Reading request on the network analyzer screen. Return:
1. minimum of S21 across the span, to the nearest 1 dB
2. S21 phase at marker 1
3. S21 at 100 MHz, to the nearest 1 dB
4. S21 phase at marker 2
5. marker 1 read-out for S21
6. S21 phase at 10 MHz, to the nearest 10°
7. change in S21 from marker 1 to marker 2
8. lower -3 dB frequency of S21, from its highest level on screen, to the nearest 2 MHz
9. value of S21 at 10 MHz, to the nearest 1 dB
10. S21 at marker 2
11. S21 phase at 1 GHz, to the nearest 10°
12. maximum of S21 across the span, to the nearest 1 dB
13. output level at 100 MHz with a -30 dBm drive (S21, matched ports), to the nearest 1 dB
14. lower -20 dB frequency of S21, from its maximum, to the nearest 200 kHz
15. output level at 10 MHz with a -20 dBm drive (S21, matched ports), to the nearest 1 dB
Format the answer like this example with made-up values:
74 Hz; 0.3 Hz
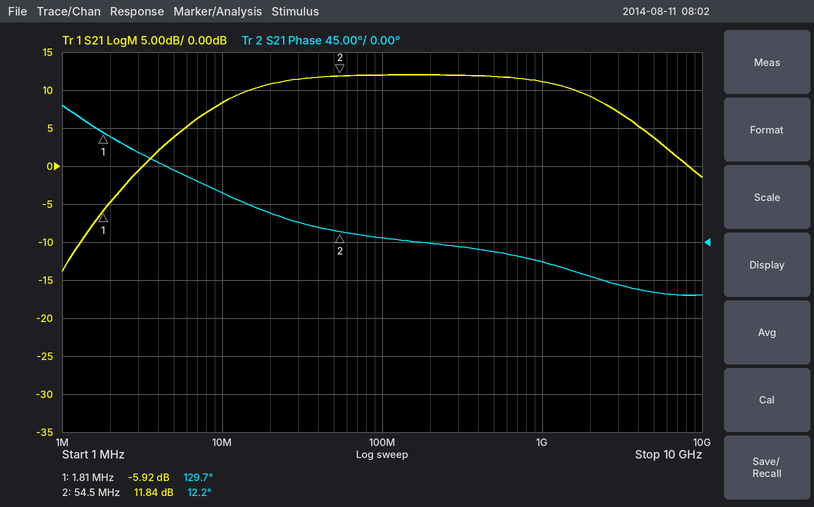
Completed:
-14 dB; 129.7°; 12 dB; 12.2°; -5.92 dB; 60°; 17.76 dB; 12 MHz; 8 dB; 11.84 dB; -20°; 12 dB; -18 dBm; 1.6 MHz; -12 dBm
